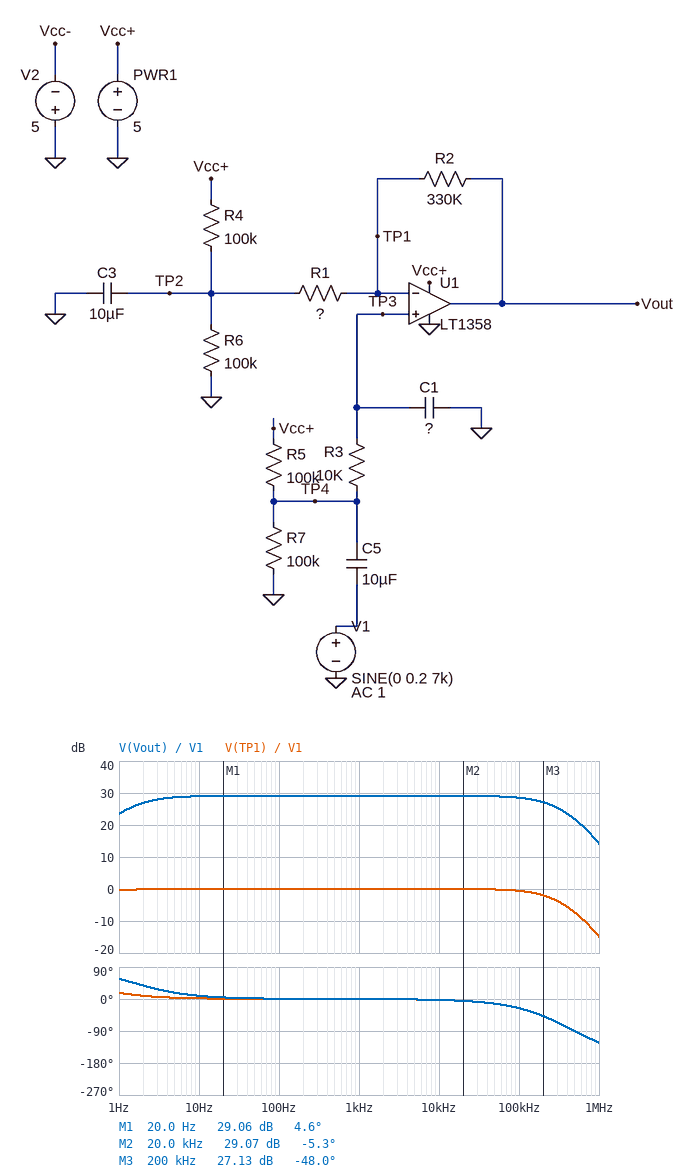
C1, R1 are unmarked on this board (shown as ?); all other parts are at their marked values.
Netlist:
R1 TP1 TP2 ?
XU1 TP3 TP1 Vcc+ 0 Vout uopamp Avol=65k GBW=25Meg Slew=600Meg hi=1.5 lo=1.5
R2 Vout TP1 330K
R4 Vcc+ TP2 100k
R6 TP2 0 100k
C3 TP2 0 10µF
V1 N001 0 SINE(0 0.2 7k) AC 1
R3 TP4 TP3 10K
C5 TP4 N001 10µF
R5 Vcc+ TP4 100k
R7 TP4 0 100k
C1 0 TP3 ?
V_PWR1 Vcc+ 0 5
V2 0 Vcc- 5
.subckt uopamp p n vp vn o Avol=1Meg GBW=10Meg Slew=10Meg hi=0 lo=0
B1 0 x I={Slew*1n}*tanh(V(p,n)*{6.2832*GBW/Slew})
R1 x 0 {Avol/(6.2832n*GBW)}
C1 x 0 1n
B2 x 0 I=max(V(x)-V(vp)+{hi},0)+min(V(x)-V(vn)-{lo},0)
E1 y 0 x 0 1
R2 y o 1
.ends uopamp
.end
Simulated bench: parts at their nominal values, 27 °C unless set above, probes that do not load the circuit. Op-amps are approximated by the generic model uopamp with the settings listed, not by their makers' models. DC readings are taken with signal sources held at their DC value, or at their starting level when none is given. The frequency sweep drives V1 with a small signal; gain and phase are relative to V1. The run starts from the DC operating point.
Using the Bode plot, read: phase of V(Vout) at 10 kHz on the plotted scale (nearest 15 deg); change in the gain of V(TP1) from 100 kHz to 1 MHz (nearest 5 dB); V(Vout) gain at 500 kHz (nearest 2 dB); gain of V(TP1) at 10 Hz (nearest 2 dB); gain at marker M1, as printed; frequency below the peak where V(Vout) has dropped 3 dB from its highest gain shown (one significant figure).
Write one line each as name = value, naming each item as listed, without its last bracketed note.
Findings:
phase of V(Vout) at 10 kHz on the plotted scale = 0 deg
change in the gain of V(TP1) from 100 kHz to 1 MHz = -15 dB
V(Vout) gain at 500 kHz = 22 dB
gain of V(TP1) at 10 Hz = 0 dB
gain at marker M1, as printed = 29.06 dB
frequency below the peak where V(Vout) has dropped 3 dB from its highest gain shown = 2 Hz
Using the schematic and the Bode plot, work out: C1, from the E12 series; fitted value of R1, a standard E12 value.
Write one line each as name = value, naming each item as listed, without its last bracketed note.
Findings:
C1, from the E12 series = 56 pF
fitted value of R1, a standard E12 value = 12 kΩ
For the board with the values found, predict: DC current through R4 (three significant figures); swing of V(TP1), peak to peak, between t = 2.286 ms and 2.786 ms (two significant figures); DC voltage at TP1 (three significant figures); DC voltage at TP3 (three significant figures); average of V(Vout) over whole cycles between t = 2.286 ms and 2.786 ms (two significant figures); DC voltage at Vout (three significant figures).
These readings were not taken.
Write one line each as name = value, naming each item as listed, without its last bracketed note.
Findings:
DC current through R4 = 25.0 µA
swing of V(TP1), peak to peak, between t = 2.286 ms and 2.786 ms = 72 mV
DC voltage at TP1 = 2.50 V
DC voltage at TP3 = 2.50 V
average of V(Vout) over whole cycles between t = 2.286 ms and 2.786 ms = 2.5 V
DC voltage at Vout = 2.50 V
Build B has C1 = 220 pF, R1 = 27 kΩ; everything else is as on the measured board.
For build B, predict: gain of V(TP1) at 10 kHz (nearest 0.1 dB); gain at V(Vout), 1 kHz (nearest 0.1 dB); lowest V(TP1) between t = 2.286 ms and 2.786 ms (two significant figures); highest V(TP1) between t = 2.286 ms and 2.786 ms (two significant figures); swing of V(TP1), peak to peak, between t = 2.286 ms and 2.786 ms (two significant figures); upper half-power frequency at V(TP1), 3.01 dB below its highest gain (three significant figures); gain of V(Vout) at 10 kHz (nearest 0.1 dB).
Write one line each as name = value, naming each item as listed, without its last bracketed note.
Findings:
gain of V(TP1) at 10 kHz = -0.1 dB
gain at V(Vout), 1 kHz = 22.4 dB
lowest V(TP1) between t = 2.286 ms and 2.786 ms = 2.4 V
highest V(TP1) between t = 2.286 ms and 2.786 ms = 2.6 V
swing of V(TP1), peak to peak, between t = 2.286 ms and 2.786 ms = 150 mV
upper half-power frequency at V(TP1), 3.01 dB below its highest gain = 72.2 kHz
gain of V(Vout) at 10 kHz = 22.3 dB
